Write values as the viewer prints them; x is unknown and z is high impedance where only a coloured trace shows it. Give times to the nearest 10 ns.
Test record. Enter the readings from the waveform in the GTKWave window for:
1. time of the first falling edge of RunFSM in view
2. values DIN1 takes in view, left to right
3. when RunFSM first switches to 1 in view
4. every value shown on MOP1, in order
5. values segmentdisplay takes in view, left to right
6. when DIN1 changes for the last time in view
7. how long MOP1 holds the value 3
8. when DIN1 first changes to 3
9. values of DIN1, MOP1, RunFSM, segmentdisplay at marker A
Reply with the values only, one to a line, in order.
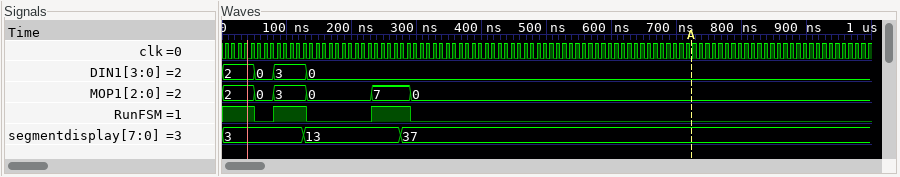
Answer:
50 ns
2, 0, 3, 0
80 ns
2, 0, 3, 0, 7, 0
3, 13, 37
130 ns
50 ns
80 ns
DIN1=0, MOP1=0, RunFSM=0, segmentdisplay=37
